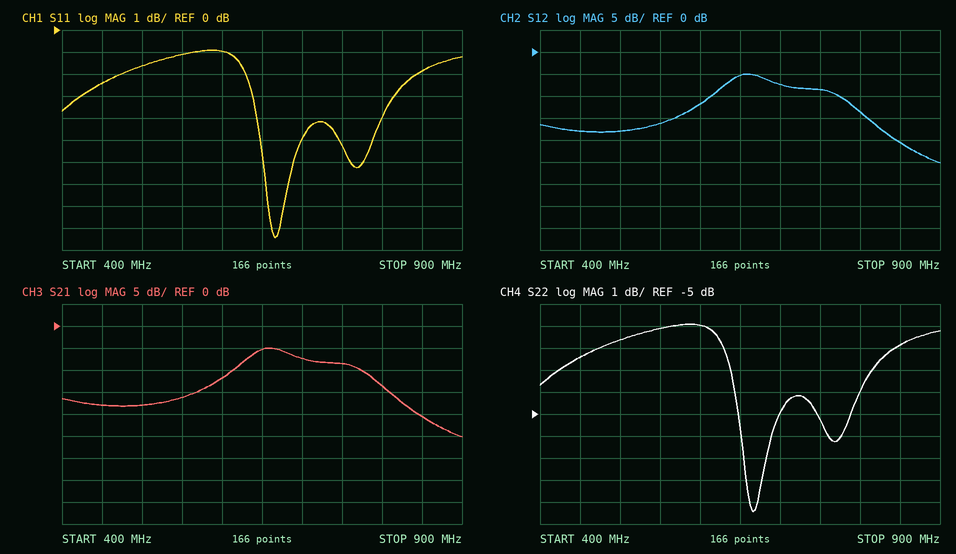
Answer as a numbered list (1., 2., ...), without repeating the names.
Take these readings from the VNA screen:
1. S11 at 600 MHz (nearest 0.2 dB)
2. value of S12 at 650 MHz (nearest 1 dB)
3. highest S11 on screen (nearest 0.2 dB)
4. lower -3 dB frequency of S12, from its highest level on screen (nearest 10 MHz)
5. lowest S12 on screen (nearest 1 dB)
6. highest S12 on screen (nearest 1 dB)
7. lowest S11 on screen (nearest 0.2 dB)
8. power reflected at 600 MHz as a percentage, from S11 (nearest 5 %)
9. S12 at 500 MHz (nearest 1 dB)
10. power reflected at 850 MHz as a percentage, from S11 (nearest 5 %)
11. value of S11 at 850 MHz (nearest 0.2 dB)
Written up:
1. -1.0 dB
2. -5 dB
3. -1.0 dB
4. 630 MHz
5. -25 dB
6. -5 dB
7. -9.4 dB
8. 80 %
9. -18 dB
10. 65 %
11. -1.8 dB
